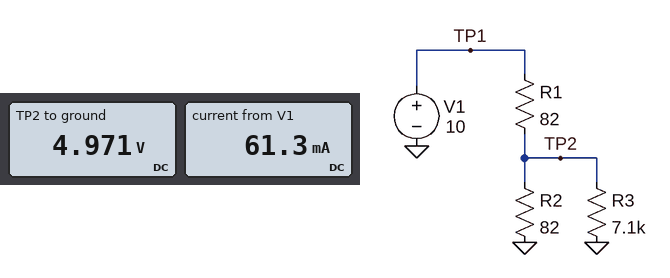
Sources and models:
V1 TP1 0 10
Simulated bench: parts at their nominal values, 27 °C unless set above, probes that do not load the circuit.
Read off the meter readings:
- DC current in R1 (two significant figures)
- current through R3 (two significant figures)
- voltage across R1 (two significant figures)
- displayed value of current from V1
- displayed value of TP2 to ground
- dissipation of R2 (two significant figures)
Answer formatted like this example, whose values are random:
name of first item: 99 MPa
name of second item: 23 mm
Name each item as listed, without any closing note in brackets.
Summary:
DC current in R1: 61 mA
current through R3: 700 µA
voltage across R1: 5.0 V
displayed value of current from V1: 61.3 mA
displayed value of TP2 to ground: 4.971 V
dissipation of R2: 300 mW
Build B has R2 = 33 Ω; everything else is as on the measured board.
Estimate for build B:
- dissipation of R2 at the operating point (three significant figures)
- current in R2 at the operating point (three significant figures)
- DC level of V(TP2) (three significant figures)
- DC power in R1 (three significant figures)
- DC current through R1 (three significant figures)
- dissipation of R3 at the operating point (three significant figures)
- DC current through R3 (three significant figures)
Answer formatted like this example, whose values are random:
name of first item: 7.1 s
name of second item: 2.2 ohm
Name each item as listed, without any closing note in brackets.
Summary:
dissipation of R2 at the operating point: 248 mW
current in R2 at the operating point: 86.7 mA
DC level of V(TP2): 2.86 V
DC power in R1: 622 mW
DC current through R1: 87.1 mA
dissipation of R3 at the operating point: 1.15 mW
DC current through R3: 403 µA
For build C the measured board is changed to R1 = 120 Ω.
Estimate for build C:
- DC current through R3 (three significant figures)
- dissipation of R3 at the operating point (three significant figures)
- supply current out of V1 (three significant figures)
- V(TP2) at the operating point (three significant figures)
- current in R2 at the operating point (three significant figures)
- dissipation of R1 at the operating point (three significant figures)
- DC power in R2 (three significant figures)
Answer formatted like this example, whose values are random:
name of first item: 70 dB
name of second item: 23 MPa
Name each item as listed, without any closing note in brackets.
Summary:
DC current through R3: 568 µA
dissipation of R3 at the operating point: 2.29 mW
supply current out of V1: 49.7 mA
V(TP2) at the operating point: 4.03 V
current in R2 at the operating point: 49.2 mA
dissipation of R1 at the operating point: 297 mW
DC power in R2: 198 mW
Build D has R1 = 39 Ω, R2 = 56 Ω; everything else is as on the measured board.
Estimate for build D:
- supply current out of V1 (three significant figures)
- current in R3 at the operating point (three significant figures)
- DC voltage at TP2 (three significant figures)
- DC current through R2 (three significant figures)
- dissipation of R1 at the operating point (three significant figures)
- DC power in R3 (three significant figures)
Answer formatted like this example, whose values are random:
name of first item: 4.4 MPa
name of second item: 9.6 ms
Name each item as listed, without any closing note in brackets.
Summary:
supply current out of V1: 106 mA
current in R3 at the operating point: 828 µA
DC voltage at TP2: 5.88 V
DC current through R2: 105 mA
dissipation of R1 at the operating point: 436 mW
DC power in R3: 4.86 mW
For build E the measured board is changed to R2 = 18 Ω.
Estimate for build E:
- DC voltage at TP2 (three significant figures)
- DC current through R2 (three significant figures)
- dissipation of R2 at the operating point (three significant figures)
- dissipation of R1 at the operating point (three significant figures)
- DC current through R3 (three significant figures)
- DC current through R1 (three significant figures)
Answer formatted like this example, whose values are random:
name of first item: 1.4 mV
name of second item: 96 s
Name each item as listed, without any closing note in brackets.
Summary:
DC voltage at TP2: 1.80 V
DC current through R2: 99.8 mA
dissipation of R2 at the operating point: 179 mW
dissipation of R1 at the operating point: 821 mW
DC current through R3: 253 µA
DC current through R1: 100 mA
